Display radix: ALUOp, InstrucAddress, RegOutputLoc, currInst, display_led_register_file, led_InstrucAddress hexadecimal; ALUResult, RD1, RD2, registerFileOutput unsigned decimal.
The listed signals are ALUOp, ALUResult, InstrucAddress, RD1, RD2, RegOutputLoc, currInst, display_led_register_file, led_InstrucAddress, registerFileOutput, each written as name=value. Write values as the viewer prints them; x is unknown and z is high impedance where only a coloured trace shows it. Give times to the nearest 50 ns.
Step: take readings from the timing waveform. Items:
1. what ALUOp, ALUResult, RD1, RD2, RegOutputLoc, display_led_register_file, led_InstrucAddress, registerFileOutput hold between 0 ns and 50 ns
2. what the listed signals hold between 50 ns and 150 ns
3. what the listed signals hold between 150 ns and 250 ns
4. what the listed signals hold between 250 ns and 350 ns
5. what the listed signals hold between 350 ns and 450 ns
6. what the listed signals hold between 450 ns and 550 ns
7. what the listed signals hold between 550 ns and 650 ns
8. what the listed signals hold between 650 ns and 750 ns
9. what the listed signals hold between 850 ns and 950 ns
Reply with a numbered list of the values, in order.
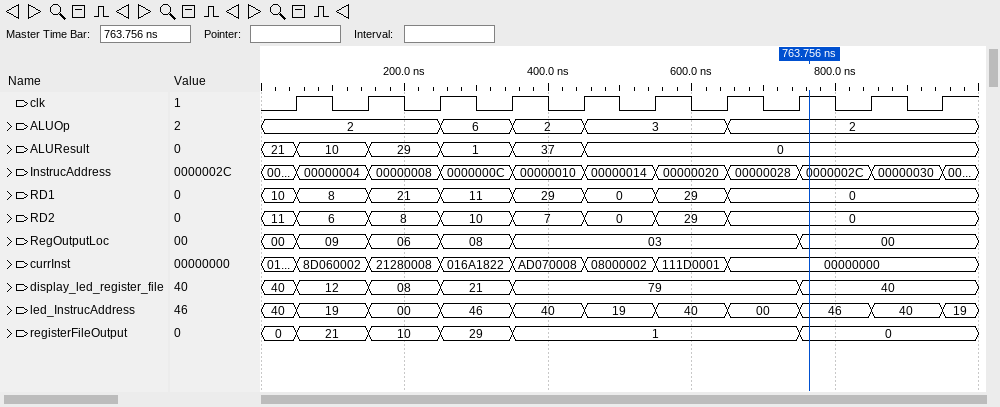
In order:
1. ALUOp=2, ALUResult=21, RD1=10, RD2=11, RegOutputLoc=00, display_led_register_file=40, led_InstrucAddress=40, registerFileOutput=0
2. ALUOp=2, ALUResult=10, InstrucAddress=00000004, RD1=8, RD2=6, RegOutputLoc=09, currInst=8D060002, display_led_register_file=12, led_InstrucAddress=19, registerFileOutput=21
3. ALUOp=2, ALUResult=29, InstrucAddress=00000008, RD1=21, RD2=8, RegOutputLoc=06, currInst=21280008, display_led_register_file=08, led_InstrucAddress=00, registerFileOutput=10
4. ALUOp=6, ALUResult=1, InstrucAddress=0000000C, RD1=11, RD2=10, RegOutputLoc=08, currInst=016A1822, display_led_register_file=21, led_InstrucAddress=46, registerFileOutput=29
5. ALUOp=2, ALUResult=37, InstrucAddress=00000010, RD1=29, RD2=7, RegOutputLoc=03, currInst=AD070008, display_led_register_file=79, led_InstrucAddress=40, registerFileOutput=1
6. ALUOp=3, ALUResult=0, InstrucAddress=00000014, RD1=0, RD2=0, RegOutputLoc=03, currInst=08000002, display_led_register_file=79, led_InstrucAddress=19, registerFileOutput=1
7. ALUOp=3, ALUResult=0, InstrucAddress=00000020, RD1=29, RD2=29, RegOutputLoc=03, currInst=111D0001, display_led_register_file=79, led_InstrucAddress=40, registerFileOutput=1
8. ALUOp=2, ALUResult=0, InstrucAddress=00000028, RD1=0, RD2=0, RegOutputLoc=03, currInst=00000000, display_led_register_file=79, led_InstrucAddress=00, registerFileOutput=1
9. ALUOp=2, ALUResult=0, InstrucAddress=00000030, RD1=0, RD2=0, RegOutputLoc=00, currInst=00000000, display_led_register_file=40, led_InstrucAddress=40, registerFileOutput=0
